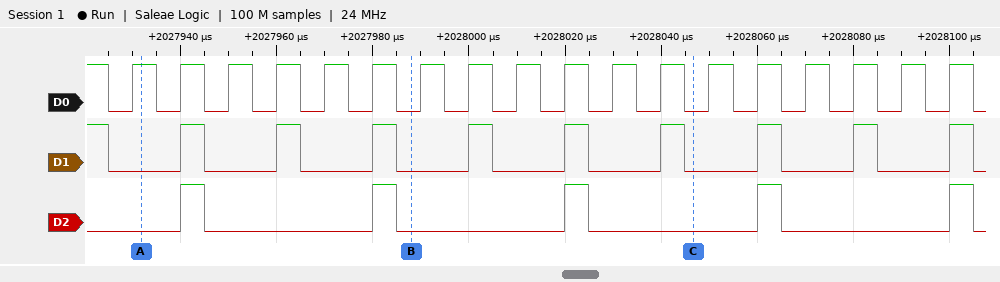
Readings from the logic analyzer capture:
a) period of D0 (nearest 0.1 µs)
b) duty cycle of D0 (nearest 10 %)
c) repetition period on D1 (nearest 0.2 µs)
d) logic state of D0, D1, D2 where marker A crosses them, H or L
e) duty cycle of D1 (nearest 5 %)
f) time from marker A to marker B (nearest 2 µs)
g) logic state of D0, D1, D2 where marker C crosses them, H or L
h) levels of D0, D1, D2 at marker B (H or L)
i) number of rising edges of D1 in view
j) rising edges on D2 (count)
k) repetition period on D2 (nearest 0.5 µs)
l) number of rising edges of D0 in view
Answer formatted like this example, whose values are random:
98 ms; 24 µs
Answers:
10 µs; 50 %; 20 µs; D0=H, D1=L, D2=L; 25 %; 56 µs; D0=L, D1=L, D2=L; D0=L, D1=L, D2=L; 9; 5; 40 µs; 18
